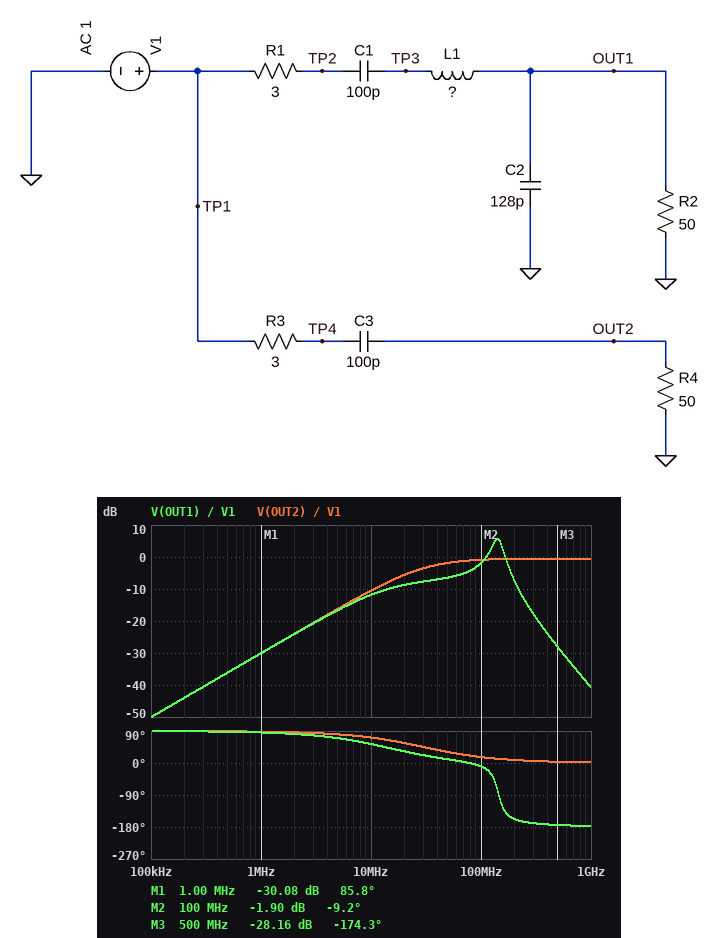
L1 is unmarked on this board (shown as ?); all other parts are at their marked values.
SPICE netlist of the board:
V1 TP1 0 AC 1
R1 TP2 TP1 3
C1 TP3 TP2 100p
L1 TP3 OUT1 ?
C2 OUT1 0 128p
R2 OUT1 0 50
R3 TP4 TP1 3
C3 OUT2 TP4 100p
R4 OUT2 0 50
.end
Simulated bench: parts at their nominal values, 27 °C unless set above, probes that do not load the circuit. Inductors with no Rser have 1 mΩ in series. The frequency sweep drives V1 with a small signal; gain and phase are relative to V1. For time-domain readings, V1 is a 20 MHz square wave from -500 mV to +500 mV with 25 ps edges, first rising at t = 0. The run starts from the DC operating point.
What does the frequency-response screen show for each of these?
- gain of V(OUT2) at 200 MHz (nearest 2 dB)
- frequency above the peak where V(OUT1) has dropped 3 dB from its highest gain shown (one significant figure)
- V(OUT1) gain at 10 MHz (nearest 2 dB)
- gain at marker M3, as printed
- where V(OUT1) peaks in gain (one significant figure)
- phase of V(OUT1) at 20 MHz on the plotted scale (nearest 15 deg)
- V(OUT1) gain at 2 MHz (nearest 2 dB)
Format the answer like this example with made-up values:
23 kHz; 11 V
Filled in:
0 dB; 200 MHz; -12 dB; -28.16 dB; 100 MHz; 30 deg; -24 dB
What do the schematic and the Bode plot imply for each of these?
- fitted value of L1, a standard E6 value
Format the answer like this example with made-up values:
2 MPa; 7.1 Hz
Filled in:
22 nH
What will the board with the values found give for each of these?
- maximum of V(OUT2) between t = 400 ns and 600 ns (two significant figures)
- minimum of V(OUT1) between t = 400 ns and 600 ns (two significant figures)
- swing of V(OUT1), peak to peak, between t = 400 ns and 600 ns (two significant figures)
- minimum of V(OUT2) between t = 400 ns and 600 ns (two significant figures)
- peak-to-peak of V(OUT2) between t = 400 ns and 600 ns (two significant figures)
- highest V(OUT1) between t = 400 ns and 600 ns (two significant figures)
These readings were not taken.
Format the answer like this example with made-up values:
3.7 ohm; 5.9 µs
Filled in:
930 mV; -630 mV; 1.3 V; -930 mV; 1.9 V; 630 mV
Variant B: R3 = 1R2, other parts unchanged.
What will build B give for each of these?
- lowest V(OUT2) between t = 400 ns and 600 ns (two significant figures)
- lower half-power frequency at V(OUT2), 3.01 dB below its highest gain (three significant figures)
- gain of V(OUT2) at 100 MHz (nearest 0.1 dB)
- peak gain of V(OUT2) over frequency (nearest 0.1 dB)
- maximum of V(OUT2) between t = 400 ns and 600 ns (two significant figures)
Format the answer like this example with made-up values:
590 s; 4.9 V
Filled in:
-970 mV; 31.1 MHz; -0.6 dB; -0.2 dB; 970 mV
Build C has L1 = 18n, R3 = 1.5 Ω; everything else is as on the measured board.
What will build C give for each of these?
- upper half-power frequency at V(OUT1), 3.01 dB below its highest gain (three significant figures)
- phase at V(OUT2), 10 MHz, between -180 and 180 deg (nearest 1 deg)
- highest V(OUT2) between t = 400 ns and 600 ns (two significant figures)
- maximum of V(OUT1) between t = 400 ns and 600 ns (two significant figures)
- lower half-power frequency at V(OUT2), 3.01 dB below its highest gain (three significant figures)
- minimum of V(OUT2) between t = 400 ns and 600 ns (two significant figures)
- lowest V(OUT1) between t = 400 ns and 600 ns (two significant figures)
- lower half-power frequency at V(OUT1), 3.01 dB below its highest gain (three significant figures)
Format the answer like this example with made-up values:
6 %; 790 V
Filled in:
174 MHz; 72 deg; 960 mV; 600 mV; 30.9 MHz; -960 mV; -600 mV; 136 MHz
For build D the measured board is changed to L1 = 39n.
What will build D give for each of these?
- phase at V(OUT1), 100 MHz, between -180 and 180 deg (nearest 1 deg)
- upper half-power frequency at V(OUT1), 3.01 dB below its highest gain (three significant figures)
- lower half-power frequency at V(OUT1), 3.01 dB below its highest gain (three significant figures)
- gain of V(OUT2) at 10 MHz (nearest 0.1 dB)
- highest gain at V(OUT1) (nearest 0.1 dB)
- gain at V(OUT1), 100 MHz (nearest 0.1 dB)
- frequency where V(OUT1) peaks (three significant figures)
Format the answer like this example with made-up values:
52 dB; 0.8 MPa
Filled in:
-48 deg; 117 MHz; 93.9 MHz; -10.5 dB; 6.2 dB; 5.1 dB; 106 MHz
